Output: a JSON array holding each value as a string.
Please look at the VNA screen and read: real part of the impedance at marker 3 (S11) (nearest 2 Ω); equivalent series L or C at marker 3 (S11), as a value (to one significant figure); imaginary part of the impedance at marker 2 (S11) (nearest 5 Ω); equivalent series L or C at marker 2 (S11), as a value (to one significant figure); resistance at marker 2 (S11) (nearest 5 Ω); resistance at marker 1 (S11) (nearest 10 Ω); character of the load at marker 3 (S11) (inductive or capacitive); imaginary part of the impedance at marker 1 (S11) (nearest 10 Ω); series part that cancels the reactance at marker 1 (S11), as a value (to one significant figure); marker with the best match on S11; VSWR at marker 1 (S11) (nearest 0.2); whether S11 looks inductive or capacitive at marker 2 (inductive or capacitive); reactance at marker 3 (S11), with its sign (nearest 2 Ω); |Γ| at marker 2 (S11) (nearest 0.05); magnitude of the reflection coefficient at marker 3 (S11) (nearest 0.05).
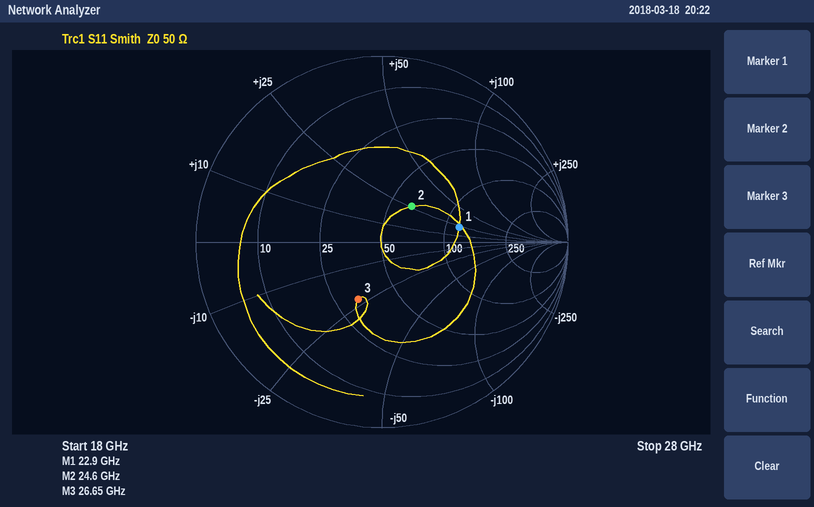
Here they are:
["32 Ω", "300 fF", "+25 Ω", "200 pH", "65 Ω", "120 Ω", "capacitive", "+20 Ω", "300 fF", "marker 2", "2.4", "inductive", "-22 Ω", "0.25", "0.35"]
